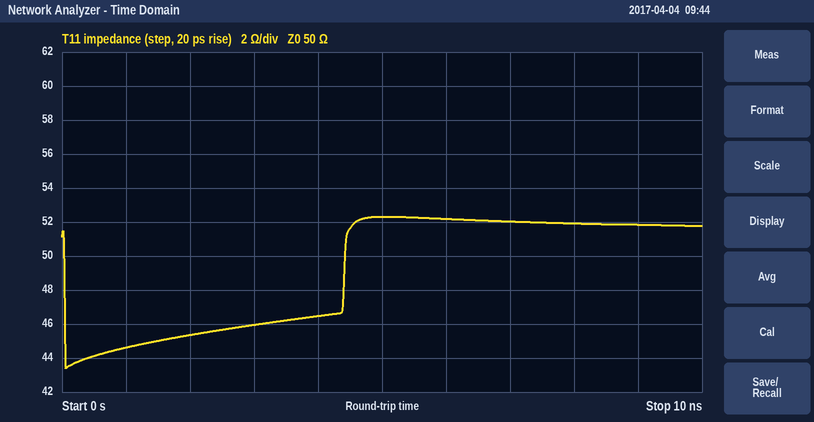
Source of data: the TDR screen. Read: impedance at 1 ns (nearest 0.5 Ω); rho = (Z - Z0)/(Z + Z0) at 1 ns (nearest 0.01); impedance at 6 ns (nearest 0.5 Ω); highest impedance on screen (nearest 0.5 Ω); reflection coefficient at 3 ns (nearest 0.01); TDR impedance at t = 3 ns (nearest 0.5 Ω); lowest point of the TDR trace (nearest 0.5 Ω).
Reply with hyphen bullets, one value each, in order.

- 44.5 Ω
- -0.06
- 52.0 Ω
- 52.5 Ω
- -0.04
- 46.0 Ω
- 43.5 Ω
